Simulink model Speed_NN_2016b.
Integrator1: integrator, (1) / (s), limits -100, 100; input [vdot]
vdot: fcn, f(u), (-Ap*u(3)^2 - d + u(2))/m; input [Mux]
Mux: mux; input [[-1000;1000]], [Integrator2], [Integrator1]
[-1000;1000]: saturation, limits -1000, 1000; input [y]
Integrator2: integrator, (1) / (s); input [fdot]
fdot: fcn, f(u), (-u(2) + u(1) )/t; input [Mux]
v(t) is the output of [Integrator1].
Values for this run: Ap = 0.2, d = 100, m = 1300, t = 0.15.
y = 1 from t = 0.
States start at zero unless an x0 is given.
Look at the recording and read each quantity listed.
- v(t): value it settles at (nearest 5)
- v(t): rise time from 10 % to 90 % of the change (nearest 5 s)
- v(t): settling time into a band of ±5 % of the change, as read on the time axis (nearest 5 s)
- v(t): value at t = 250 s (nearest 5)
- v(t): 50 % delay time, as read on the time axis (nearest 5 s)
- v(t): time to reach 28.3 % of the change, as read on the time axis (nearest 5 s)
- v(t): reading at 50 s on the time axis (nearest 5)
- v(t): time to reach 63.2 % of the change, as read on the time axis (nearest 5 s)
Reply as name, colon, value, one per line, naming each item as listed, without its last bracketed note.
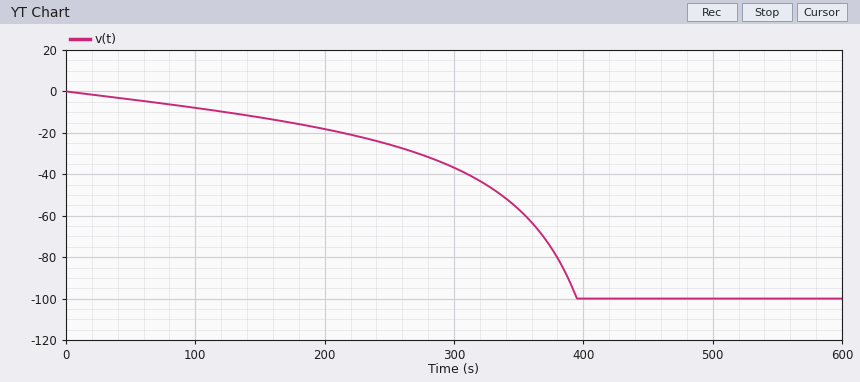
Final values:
v(t): value it settles at: -100
v(t): rise time from 10 % to 90 % of the change: 265 s
v(t): settling time into a band of ±5 % of the change, as read on the time axis: 390 s
v(t): value at t = 250 s: -25
v(t): 50 % delay time, as read on the time axis: 335 s
v(t): time to reach 28.3 % of the change, as read on the time axis: 265 s
v(t): reading at 50 s on the time axis: -5
v(t): time to reach 63.2 % of the change, as read on the time axis: 360 s
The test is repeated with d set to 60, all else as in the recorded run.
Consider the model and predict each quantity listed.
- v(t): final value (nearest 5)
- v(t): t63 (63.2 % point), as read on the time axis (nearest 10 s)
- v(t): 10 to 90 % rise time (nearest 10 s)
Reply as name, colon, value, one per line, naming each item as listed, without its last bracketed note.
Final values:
v(t): final value: -100
v(t): t63 (63.2 % point), as read on the time axis: 490 s
v(t): 10 to 90 % rise time: 320 s
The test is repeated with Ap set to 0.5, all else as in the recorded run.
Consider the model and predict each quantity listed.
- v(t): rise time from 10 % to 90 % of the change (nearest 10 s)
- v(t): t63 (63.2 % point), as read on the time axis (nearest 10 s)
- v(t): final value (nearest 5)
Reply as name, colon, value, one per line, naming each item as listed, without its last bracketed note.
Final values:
v(t): rise time from 10 % to 90 % of the change: 150 s
v(t): t63 (63.2 % point), as read on the time axis: 250 s
v(t): final value: -100
